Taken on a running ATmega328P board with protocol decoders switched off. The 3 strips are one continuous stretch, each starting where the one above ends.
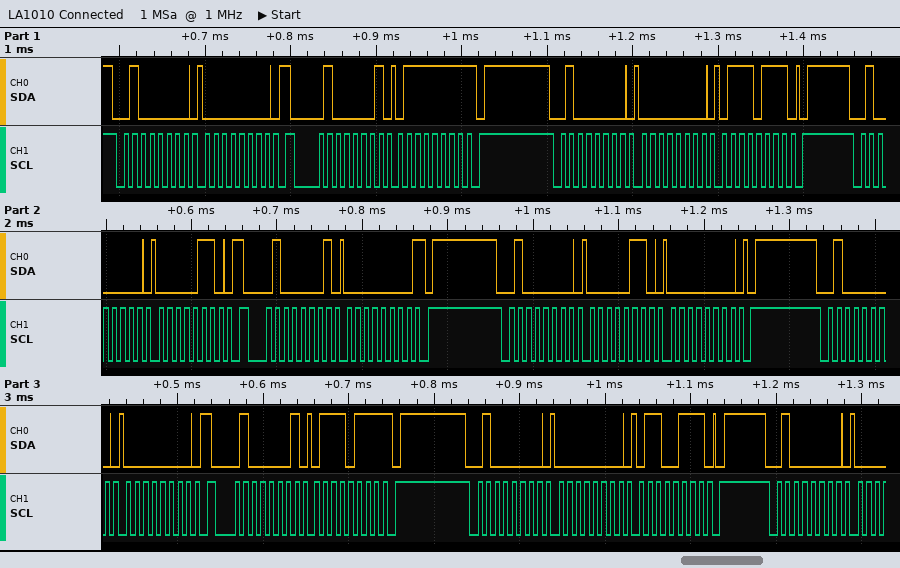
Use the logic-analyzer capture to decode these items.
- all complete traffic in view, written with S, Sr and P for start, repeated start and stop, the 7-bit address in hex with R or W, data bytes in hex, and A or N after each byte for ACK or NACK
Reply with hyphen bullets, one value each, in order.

- S 20W A 00 A Sr 20R A 7F N P S 20W A 00 A 77 A P S 20W A 06 A Sr 20R A 00 N P S 20W A 06 A 00 A P S 20W A 00 A Sr 20R A 77 N P S 20W A 00 A 67 A P S 20W A
